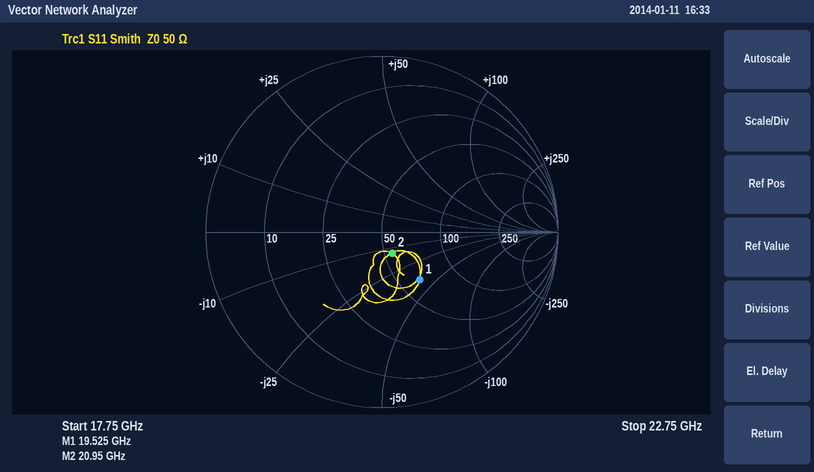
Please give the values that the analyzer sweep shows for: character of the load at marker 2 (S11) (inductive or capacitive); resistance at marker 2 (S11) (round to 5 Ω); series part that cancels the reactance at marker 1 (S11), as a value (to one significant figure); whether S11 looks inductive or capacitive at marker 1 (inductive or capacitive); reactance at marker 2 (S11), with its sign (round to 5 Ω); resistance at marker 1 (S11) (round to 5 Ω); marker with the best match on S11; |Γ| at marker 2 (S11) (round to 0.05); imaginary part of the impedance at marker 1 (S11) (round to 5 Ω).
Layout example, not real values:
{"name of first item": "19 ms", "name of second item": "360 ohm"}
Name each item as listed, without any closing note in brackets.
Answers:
{"character of the load at marker 2 (S11)": "capacitive", "resistance at marker 2 (S11)": "55 Ω", "series part that cancels the reactance at marker 1 (S11), as a value": "300 pH", "whether S11 looks inductive or capacitive at marker 1": "capacitive", "reactance at marker 2 (S11), with its sign": "-15 Ω", "resistance at marker 1 (S11)": "65 Ω", "marker with the best match on S11": "marker 2", "|Γ| at marker 2 (S11)": "0.15", "imaginary part of the impedance at marker 1 (S11)": "-40 Ω"}
